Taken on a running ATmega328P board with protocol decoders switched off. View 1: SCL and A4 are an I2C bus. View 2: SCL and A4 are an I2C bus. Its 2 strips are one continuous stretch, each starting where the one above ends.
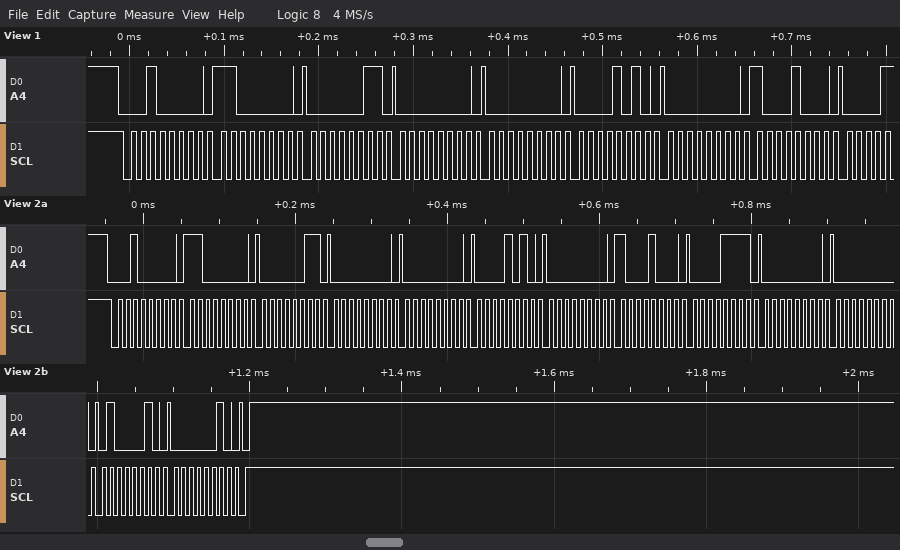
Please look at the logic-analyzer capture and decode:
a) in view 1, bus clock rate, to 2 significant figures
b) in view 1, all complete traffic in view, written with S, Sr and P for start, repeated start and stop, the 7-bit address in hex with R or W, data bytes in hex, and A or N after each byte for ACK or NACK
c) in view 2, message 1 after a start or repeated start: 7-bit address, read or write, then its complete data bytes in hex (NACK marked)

100 kHz
S 10W A C0 A 03 A 00 A 00 A 0A A 00 A 88 A
0x10 write: C0 03 00 00 0A 00 88 0F 00 00 42 02
